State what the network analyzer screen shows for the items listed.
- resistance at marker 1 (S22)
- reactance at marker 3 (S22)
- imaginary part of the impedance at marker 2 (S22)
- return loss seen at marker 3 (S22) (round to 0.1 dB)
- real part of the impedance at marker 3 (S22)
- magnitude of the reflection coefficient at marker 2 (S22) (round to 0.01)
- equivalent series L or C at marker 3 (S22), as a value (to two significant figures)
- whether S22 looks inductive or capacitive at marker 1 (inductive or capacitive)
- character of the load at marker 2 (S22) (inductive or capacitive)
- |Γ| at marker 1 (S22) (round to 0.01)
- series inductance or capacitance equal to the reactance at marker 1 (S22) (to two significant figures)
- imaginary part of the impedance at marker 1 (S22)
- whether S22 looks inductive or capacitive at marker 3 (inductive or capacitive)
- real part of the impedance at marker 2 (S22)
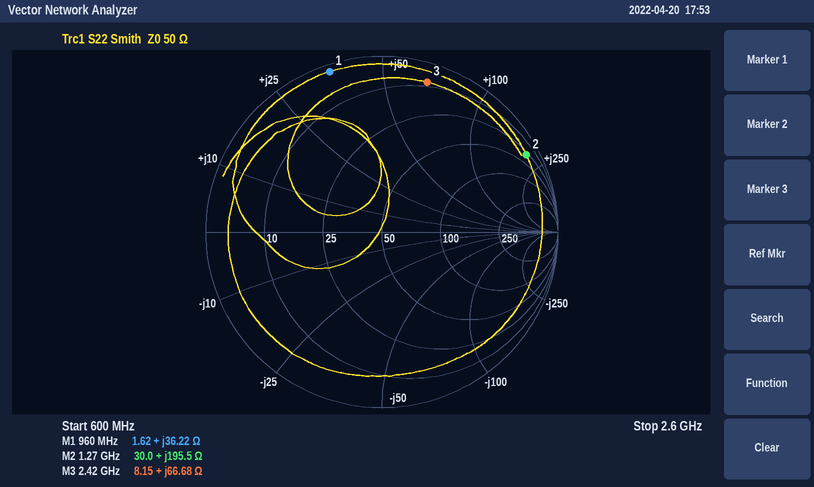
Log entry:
1.62 Ω
+66.68 Ω
+195.5 Ω
1.0 dB
8.15 Ω
0.93
4.4 nH
inductive
inductive
0.96
6.0 nH
+36.22 Ω
inductive
30.0 Ω
